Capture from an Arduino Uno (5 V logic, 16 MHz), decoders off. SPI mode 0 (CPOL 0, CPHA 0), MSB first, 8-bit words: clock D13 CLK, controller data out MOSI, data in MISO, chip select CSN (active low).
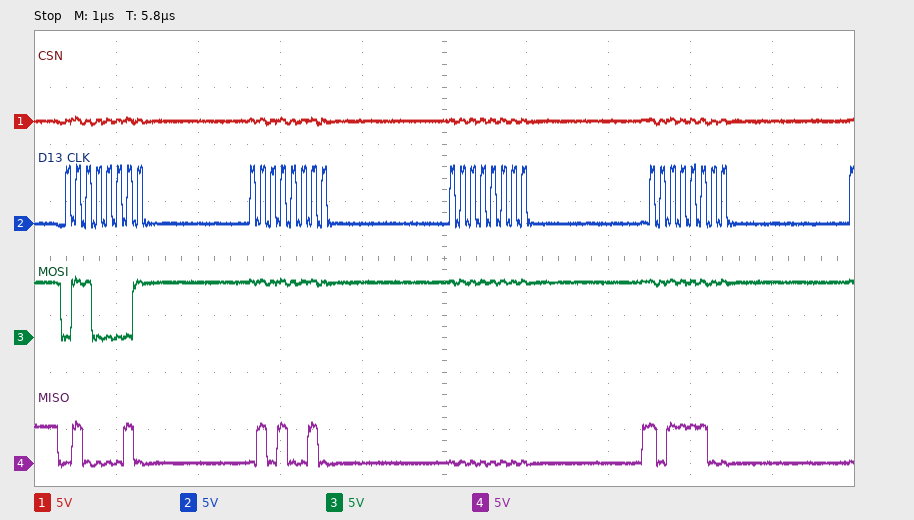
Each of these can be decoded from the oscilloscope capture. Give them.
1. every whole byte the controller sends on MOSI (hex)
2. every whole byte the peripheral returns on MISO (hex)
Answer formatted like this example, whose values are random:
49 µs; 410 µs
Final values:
61 FF FF FF; 42 52 00 BC
